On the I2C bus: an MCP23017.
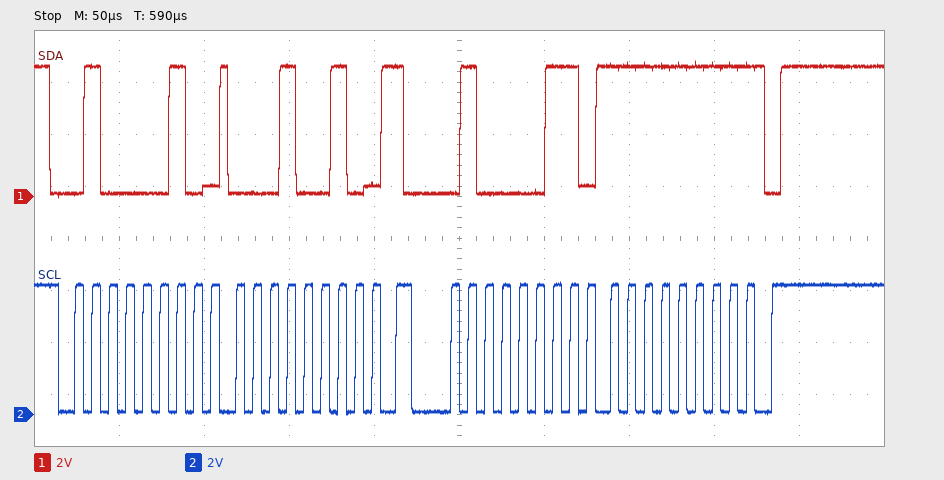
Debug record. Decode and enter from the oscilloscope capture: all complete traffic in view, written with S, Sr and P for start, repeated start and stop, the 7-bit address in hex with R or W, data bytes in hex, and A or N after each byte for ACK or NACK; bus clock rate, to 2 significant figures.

S 21W A 12 A Sr 21R A FF N P
100 kHz
